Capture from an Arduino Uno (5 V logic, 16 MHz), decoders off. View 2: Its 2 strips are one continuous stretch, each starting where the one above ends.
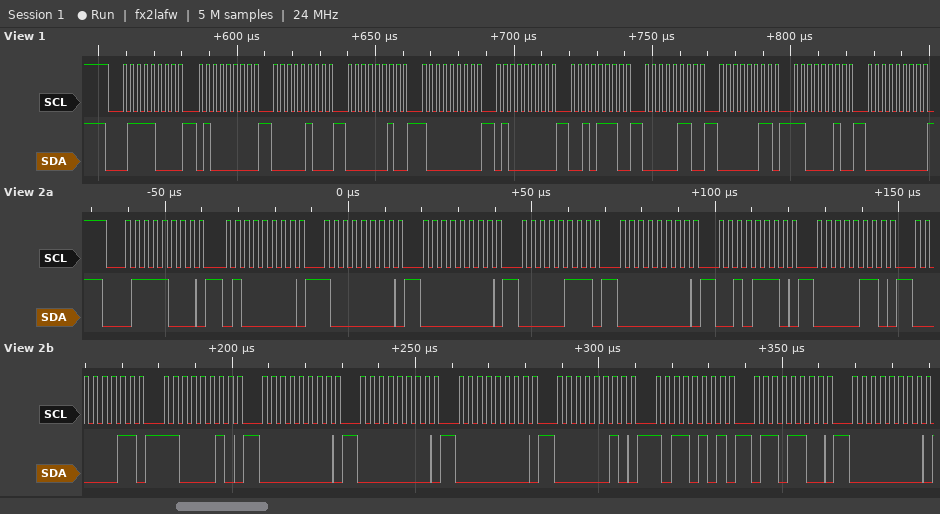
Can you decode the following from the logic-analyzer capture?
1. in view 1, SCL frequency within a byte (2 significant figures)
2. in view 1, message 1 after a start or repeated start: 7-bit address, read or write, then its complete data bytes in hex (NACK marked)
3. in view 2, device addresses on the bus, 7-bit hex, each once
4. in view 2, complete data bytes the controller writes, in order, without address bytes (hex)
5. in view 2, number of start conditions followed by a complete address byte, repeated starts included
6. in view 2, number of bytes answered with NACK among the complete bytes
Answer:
400 kHz
0x3C write: 40 04 02 80 40 2E 06 03 C2 00
0x3C
40 80 00 07 00 2E 06 03 C2 00 00 00 02 B5 6C 00
1
0
